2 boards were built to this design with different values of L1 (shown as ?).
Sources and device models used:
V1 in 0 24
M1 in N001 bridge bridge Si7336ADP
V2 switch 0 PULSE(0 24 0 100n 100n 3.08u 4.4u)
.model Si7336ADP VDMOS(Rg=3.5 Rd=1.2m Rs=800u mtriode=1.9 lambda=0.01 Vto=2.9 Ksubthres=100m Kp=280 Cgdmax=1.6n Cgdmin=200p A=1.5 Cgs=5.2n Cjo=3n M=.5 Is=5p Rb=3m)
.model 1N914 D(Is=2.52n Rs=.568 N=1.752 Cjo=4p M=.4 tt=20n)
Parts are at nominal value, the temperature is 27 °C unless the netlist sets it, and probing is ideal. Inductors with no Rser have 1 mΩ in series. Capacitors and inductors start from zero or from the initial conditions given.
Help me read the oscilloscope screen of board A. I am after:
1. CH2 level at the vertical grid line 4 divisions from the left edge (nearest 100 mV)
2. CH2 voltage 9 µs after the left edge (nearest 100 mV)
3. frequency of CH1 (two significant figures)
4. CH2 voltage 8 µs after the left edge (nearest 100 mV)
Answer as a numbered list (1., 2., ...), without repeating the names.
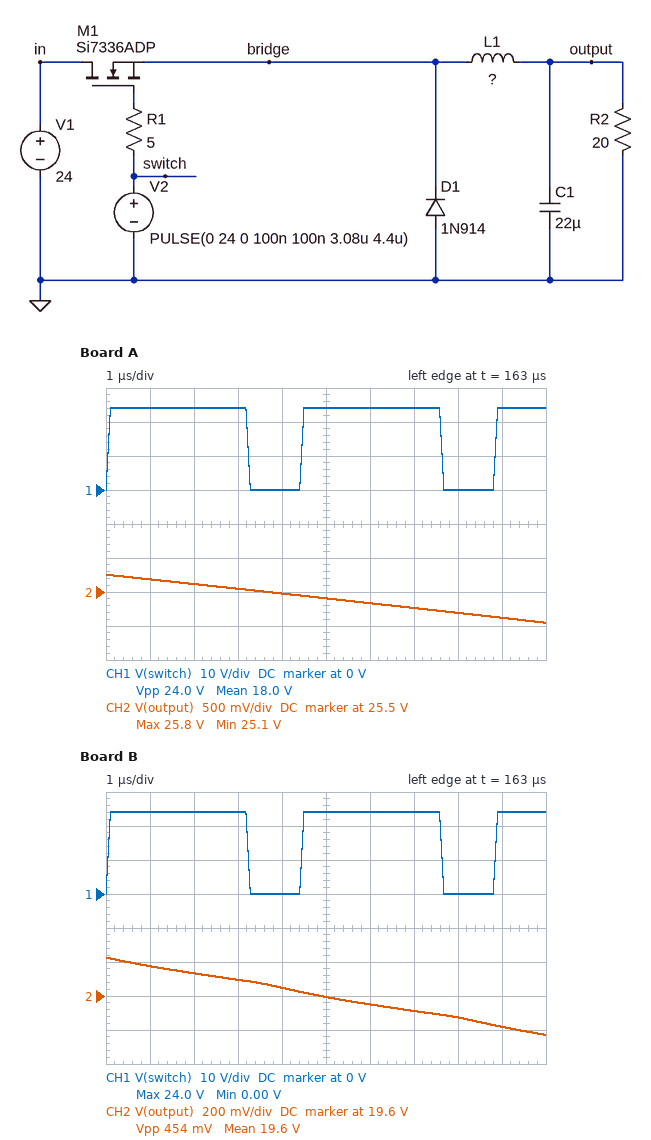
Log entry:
1. 25.5 V
2. 25.1 V
3. 230 kHz
4. 25.2 V
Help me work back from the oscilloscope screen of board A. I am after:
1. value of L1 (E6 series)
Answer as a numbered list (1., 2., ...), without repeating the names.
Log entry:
1. 100 µH
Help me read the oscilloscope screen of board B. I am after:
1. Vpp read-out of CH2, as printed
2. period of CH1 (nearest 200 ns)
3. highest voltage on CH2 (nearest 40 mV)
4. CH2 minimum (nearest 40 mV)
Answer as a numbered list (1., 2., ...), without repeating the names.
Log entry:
1. 454 mV
2. 4.4 µs
3. 19.84 V
4. 19.36 V
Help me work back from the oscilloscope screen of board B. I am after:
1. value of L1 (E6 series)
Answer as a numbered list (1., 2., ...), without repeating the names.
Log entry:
1. 22 µH
